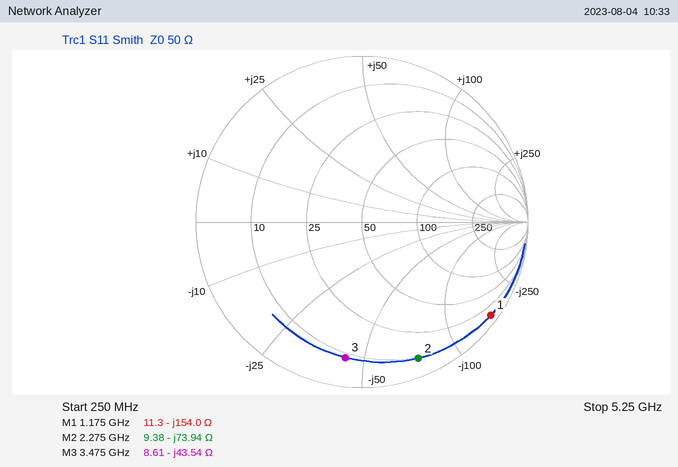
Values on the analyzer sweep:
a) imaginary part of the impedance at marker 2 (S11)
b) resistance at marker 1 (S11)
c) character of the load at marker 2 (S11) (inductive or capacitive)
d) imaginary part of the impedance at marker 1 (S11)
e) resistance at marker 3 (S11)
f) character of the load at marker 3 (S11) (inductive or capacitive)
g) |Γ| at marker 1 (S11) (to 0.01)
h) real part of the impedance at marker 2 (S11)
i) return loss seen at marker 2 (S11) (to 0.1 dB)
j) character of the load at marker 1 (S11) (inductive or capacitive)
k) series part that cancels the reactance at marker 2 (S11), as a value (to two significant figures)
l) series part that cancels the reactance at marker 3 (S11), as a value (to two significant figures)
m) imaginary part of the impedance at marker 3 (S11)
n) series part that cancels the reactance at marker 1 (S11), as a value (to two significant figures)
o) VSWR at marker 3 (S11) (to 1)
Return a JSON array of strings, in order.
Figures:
["-73.94 Ω", "11.3 Ω", "capacitive", "-154.0 Ω", "8.61 Ω", "capacitive", "0.96", "9.38 Ω", "1.0 dB", "capacitive", "5.2 nH", "2.0 nH", "-43.54 Ω", "21 nH", "10"]
